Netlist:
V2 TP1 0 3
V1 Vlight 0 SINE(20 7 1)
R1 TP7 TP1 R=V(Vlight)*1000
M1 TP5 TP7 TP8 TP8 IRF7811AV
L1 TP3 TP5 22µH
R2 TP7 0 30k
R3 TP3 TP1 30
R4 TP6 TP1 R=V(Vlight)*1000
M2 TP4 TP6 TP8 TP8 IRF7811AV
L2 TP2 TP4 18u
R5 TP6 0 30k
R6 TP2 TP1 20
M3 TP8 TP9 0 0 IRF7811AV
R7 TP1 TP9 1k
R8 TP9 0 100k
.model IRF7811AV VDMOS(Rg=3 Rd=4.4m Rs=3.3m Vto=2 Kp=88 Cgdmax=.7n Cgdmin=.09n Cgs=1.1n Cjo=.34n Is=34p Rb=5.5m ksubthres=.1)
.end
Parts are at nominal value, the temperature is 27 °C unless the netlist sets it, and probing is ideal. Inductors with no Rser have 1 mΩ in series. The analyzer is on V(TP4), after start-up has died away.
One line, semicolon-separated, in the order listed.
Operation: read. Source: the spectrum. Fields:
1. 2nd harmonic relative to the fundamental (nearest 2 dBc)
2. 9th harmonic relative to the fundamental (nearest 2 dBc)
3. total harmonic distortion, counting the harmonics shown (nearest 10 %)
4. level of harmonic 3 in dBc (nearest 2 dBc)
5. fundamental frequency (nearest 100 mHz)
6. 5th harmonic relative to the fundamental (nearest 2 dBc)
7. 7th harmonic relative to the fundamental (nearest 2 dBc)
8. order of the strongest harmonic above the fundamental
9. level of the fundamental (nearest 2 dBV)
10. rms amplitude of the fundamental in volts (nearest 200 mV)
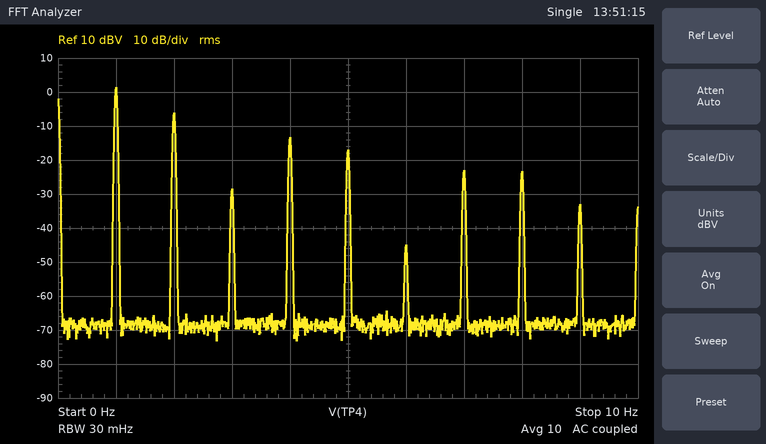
-8 dBc; -34 dBc; 50 %; -30 dBc; 1.0 Hz; -18 dBc; -24 dBc; 2; 2 dBV; 1.2 V
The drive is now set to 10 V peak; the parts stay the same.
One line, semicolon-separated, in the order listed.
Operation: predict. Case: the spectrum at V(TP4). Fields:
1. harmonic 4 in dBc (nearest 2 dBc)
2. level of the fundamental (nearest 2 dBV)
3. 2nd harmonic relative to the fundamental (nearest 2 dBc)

-14 dBc; 2 dBV; -10 dBc
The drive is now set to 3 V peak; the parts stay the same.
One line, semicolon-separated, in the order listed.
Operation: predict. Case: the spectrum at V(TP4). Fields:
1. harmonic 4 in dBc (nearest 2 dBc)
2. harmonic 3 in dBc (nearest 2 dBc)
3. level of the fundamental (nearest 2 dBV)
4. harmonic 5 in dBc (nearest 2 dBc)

-30 dBc; -18 dBc; -10 dBV; -46 dBc
